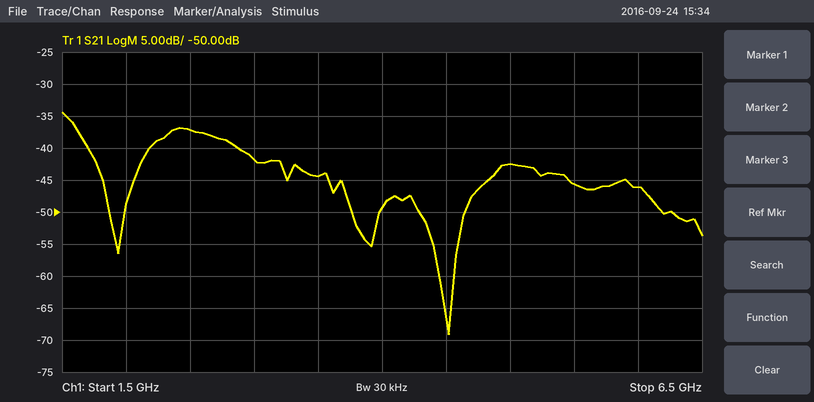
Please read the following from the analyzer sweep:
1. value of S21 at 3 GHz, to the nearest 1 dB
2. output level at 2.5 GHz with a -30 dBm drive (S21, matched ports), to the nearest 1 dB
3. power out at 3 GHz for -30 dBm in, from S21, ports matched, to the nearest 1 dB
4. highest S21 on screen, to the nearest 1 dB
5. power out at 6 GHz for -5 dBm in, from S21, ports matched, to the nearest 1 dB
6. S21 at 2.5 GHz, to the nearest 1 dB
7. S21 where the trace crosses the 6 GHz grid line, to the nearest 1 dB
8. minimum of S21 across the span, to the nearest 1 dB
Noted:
-42 dB
-67 dBm
-72 dBm
-34 dB
-51 dBm
-37 dB
-46 dB
-69 dB
